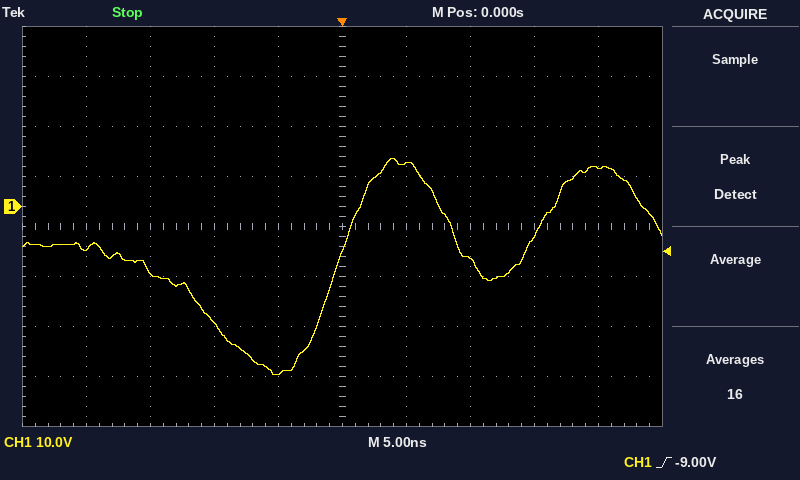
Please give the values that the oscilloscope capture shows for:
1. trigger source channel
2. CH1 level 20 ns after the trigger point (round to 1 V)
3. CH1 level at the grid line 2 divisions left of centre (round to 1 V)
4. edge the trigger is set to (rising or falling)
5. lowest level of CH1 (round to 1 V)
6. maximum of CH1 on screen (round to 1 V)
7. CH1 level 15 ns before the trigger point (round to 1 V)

CH1
8 V
-23 V
rising
-34 V
10 V
-13 V
